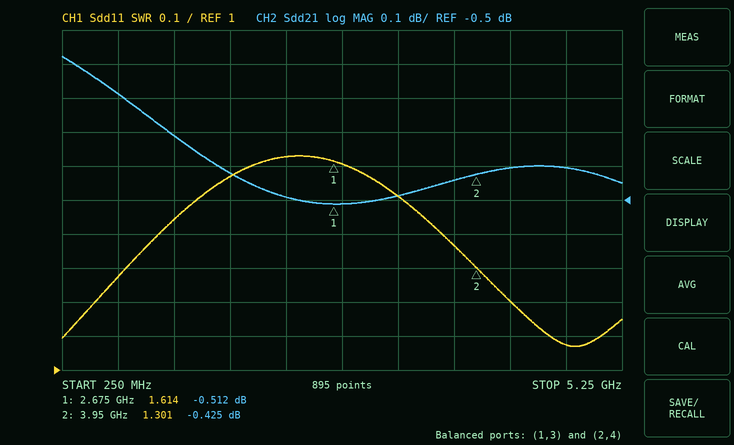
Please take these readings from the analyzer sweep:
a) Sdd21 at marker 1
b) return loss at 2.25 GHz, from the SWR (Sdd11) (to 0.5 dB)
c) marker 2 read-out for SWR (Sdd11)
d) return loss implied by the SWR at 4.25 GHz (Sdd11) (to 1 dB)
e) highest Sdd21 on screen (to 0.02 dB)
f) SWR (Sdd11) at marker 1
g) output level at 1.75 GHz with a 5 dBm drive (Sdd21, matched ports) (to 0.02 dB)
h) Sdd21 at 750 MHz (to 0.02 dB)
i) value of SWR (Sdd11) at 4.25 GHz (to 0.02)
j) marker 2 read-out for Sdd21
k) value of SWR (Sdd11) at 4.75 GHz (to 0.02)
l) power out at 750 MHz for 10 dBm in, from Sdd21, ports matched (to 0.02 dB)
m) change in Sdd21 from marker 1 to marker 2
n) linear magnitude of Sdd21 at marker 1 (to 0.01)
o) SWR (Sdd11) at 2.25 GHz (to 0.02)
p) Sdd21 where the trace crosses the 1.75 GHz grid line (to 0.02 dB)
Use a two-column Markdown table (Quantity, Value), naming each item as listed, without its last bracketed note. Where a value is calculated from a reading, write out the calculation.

| Quantity | Value |
|---|---|
| Sdd21 at marker 1 | -0.512 dB |
| return loss at 2.25 GHz, from the SWR (Sdd11) | −20 log10((1.62 − 1)/(1.62 + 1)) ≈ 12.5 dB |
| marker 2 read-out for SWR | 1.301 |
| return loss implied by the SWR at 4.25 GHz (Sdd11) | −20 log10((1.2 − 1)/(1.2 + 1)) ≈ 21 dB |
| highest Sdd21 on screen | -0.08 dB |
| SWR (Sdd11) at marker 1 | 1.614 |
| output level at 1.75 GHz with a 5 dBm drive (Sdd21, matched ports) | 5 dBm + (-0.42 dB) = 4.58 dBm |
| Sdd21 at 750 MHz | -0.18 dB |
| value of SWR (Sdd11) at 4.25 GHz | 1.20 |
| marker 2 read-out for Sdd21 | -0.425 dB |
| value of SWR (Sdd11) at 4.75 GHz | 1.08 |
| power out at 750 MHz for 10 dBm in, from Sdd21, ports matched | 10 dBm + (-0.18 dB) = 9.82 dBm |
| change in Sdd21 from marker 1 to marker 2 | -0.425 − (-0.512) = 0.087 dB |
| linear magnitude of Sdd21 at marker 1 | 10^(-0.512/20) ≈ 0.94 |
| SWR (Sdd11) at 2.25 GHz | 1.62 |
| Sdd21 where the trace crosses the 1.75 GHz grid line | -0.42 dB |
